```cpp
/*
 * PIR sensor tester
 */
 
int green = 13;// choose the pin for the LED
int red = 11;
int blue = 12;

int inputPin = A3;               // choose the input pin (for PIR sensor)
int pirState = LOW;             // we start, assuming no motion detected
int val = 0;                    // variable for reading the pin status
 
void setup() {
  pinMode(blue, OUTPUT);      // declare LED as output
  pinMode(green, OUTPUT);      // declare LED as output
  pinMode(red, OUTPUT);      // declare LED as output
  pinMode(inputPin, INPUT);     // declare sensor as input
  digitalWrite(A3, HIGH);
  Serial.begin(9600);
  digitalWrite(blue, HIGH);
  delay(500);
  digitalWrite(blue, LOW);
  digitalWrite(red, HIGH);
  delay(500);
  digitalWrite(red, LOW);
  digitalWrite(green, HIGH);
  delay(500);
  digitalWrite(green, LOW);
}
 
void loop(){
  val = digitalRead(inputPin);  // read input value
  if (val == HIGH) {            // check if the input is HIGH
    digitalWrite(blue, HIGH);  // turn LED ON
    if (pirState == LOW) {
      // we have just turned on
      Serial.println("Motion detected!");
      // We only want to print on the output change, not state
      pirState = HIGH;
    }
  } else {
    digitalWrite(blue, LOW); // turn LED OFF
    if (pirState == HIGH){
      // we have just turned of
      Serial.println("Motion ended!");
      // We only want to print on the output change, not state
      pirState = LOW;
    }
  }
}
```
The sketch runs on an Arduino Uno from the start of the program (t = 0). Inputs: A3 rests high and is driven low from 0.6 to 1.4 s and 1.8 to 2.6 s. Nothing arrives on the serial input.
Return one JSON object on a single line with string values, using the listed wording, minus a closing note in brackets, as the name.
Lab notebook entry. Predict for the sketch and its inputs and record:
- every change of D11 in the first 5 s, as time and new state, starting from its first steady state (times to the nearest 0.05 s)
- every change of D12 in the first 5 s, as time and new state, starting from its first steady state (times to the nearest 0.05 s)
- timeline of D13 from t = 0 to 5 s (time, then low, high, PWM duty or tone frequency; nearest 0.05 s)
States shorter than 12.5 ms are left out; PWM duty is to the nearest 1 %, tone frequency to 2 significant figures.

{"every change of D11 in the first 5 s, as time and new state, starting from its first steady state": "0 s low; 0.5 s high; 1 s low", "every change of D12 in the first 5 s, as time and new state, starting from its first steady state": "0 s high; 0.5 s low; 1.5 s high; 1.8 s low; 2.6 s high", "timeline of D13 from t = 0 to 5 s": "0 s low; 1 s high; 1.5 s low"}
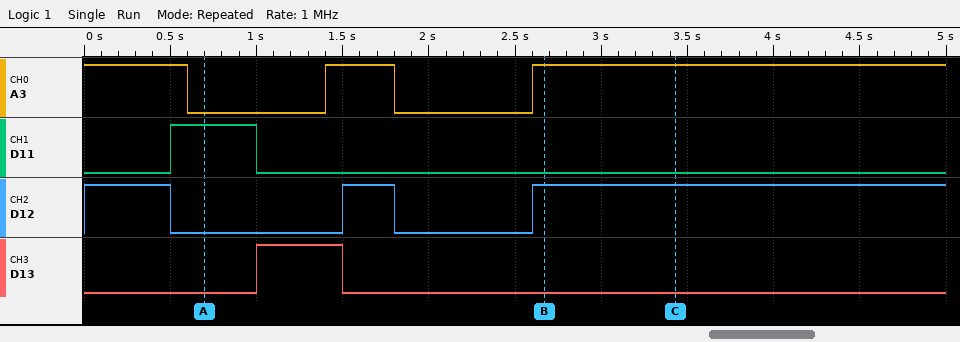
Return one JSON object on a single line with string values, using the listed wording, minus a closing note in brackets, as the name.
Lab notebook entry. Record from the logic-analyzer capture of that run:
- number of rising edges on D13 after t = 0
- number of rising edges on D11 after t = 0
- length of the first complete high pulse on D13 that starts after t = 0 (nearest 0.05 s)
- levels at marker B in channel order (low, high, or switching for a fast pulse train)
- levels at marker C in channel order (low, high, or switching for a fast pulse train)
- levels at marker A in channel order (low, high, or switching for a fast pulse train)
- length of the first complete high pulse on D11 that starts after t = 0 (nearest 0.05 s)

{"number of rising edges on D13 after t = 0": "1", "number of rising edges on D11 after t = 0": "1", "length of the first complete high pulse on D13 that starts after t = 0": "0.50 s", "levels at marker B in channel order": "A3 high, D11 low, D12 high, D13 low", "levels at marker C in channel order": "A3 high, D11 low, D12 high, D13 low", "levels at marker A in channel order": "A3 low, D11 high, D12 low, D13 low", "length of the first complete high pulse on D11 that starts after t = 0": "0.50 s"}
